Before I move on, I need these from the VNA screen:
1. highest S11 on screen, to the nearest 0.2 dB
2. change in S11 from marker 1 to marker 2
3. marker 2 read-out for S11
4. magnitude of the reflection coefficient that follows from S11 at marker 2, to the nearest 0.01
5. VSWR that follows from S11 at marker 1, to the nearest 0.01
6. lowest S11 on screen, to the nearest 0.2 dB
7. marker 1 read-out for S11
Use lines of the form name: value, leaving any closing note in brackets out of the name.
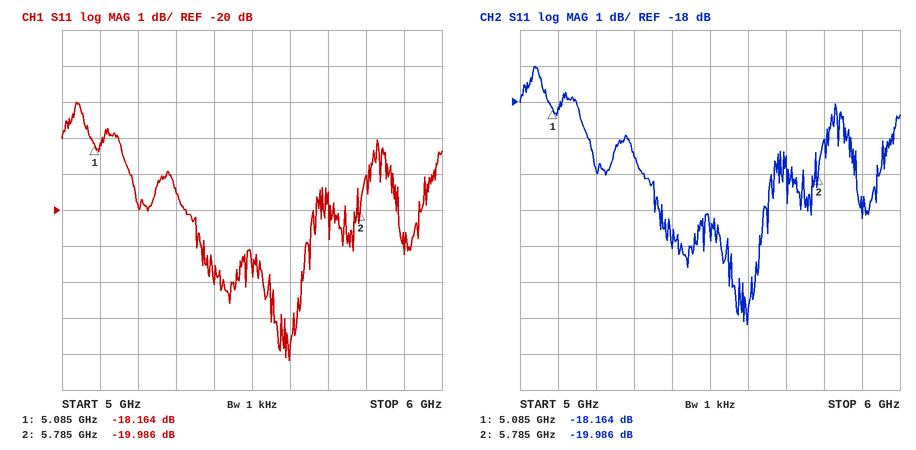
highest S11 on screen, to the nearest 0.2 dB: -17.0 dB
change in S11 from marker 1 to marker 2: -1.822 dB
marker 2 read-out for S11: -19.986 dB
magnitude of the reflection coefficient that follows from S11 at marker 2, to the nearest 0.01: 0.10
VSWR that follows from S11 at marker 1, to the nearest 0.01: 1.28
lowest S11 on screen, to the nearest 0.2 dB: -24.2 dB
marker 1 read-out for S11: -18.164 dB
